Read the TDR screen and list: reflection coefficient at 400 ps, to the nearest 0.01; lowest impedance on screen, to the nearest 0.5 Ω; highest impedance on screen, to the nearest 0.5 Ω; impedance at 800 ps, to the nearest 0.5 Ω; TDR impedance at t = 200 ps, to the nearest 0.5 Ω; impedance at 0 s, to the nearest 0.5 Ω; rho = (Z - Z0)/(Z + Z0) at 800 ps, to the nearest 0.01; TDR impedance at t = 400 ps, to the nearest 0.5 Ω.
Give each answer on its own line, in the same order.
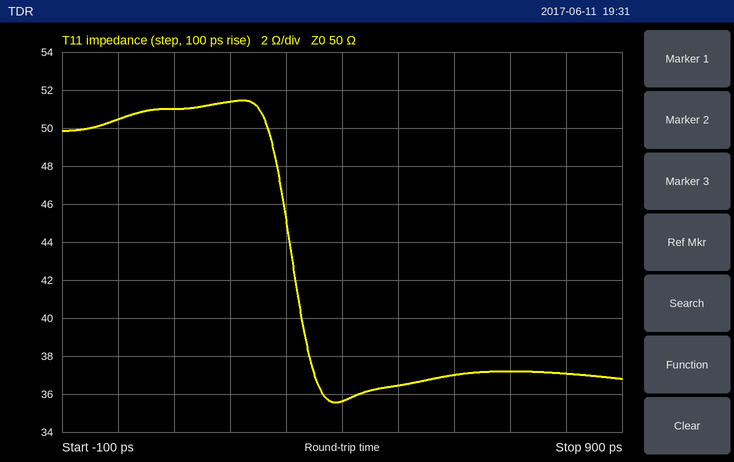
-0.17
35.5 Ω
51.5 Ω
37.0 Ω
51.5 Ω
50.5 Ω
-0.15
35.5 Ω
